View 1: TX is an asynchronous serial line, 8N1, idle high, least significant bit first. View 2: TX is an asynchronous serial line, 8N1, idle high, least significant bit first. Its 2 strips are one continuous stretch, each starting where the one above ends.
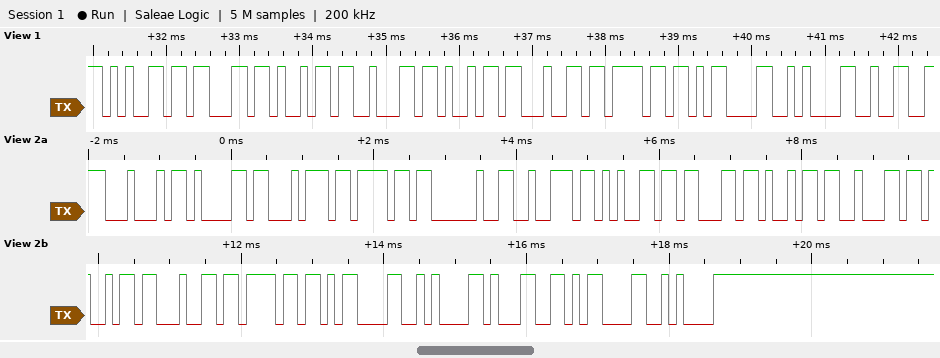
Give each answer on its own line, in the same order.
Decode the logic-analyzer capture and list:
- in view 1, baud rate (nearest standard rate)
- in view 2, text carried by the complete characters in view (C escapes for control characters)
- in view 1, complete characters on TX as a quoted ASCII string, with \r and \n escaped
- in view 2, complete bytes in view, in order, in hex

9600 baud
"Dato recibido\r\n1\r\n"
"ecibido\r\n2"
44 61 74 6F 20 72 65 63 69 62 69 64 6F 0D 0A 31 0D 0A
